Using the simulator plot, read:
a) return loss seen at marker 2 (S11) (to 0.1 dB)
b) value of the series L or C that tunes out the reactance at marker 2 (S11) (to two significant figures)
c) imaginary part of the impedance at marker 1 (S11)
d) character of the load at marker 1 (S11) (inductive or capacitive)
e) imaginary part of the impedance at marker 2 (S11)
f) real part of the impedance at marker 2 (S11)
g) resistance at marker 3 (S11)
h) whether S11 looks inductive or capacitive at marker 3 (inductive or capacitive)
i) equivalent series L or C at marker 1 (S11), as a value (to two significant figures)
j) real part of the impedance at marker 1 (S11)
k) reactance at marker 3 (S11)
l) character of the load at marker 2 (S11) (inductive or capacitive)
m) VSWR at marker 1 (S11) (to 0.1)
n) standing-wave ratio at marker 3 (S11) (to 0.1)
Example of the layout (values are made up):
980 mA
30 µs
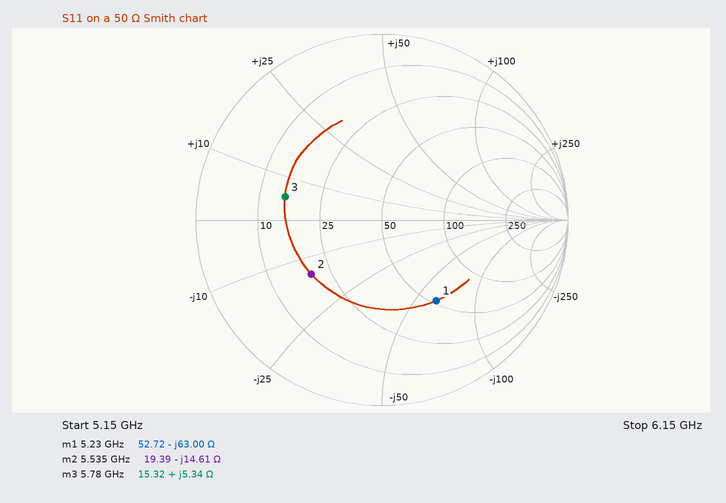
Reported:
6.4 dB
420 pH
-63.00 Ω
capacitive
-14.61 Ω
19.39 Ω
15.32 Ω
inductive
480 fF
52.72 Ω
+5.34 Ω
capacitive
3.2
3.3
